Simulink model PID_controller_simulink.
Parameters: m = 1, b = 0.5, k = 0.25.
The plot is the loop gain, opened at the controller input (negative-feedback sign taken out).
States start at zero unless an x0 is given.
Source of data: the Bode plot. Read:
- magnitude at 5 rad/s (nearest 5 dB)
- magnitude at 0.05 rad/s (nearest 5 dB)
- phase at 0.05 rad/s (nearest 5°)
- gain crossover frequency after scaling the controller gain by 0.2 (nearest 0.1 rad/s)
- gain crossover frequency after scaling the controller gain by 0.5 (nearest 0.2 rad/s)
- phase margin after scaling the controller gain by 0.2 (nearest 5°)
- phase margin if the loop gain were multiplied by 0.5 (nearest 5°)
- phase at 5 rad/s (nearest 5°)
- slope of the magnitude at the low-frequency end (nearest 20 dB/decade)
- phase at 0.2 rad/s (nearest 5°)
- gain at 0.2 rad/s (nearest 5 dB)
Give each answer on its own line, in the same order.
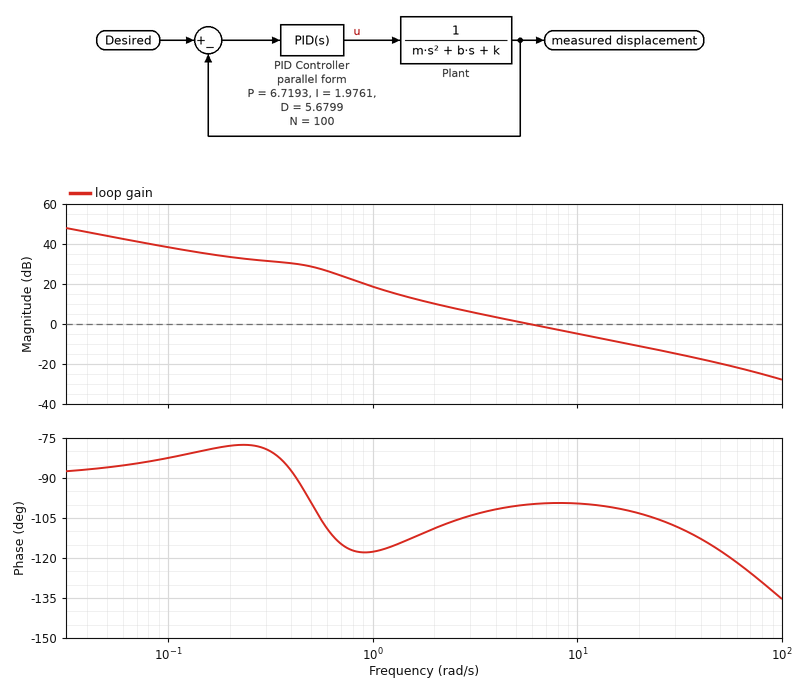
0 dB
45 dB
-85°
1.4 rad/s
3.0 rad/s
65°
75°
-100°
-20 dB/decade
-80°
35 dB
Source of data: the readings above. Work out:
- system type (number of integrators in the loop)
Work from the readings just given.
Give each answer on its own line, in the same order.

1
